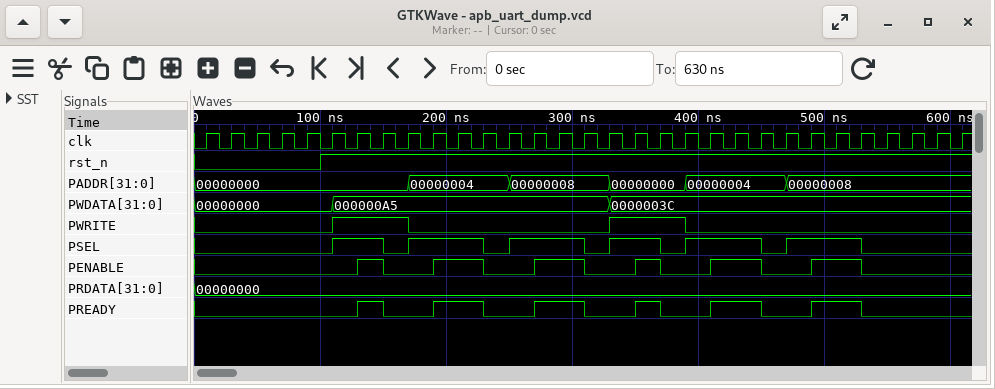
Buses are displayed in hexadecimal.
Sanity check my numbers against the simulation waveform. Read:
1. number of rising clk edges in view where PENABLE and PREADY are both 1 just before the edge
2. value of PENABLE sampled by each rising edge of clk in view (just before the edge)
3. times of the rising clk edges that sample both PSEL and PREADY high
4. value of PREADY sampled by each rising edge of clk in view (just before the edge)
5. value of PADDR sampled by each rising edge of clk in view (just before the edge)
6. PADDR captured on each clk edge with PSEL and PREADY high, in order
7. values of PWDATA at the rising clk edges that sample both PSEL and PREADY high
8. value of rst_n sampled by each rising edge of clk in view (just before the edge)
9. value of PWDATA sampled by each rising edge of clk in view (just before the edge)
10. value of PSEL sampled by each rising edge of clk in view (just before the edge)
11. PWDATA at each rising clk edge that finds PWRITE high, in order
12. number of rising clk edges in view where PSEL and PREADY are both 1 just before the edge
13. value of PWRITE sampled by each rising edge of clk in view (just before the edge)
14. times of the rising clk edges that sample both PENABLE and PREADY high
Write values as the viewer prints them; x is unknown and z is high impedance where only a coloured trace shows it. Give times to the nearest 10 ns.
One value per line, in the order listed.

10
0 0 0 0 0 0 0 1 0 0 1 1 0 0 1 1 0 0 1 0 0 1 1 0 0 1 1 0 0 0 0
150 ns, 210 ns, 230 ns, 290 ns, 310 ns, 370 ns, 430 ns, 450 ns, 510 ns, 530 ns
0 0 0 0 0 0 0 1 0 0 1 1 0 0 1 1 0 0 1 0 0 1 1 0 0 1 1 0 0 0 0
00000000, 00000000, 00000000, 00000000, 00000000, 00000000, 00000000, 00000000, 00000000, 00000004, 00000004, 00000004, 00000004, 00000008, 00000008, 00000008, 00000008, 00000000, 00000000, 00000000, 00000004, 00000004, 00000004, 00000004, 00000008, 00000008, 00000008, 00000008, 00000008, 00000008, 00000008
00000000, 00000004, 00000004, 00000008, 00000008, 00000000, 00000004, 00000004, 00000008, 00000008
000000A5, 000000A5, 000000A5, 000000A5, 000000A5, 0000003C, 0000003C, 0000003C, 0000003C, 0000003C
0 0 0 0 0 1 1 1 1 1 1 1 1 1 1 1 1 1 1 1 1 1 1 1 1 1 1 1 1 1 1
00000000, 00000000, 00000000, 00000000, 00000000, 00000000, 000000A5, 000000A5, 000000A5, 000000A5, 000000A5, 000000A5, 000000A5, 000000A5, 000000A5, 000000A5, 000000A5, 0000003C, 0000003C, 0000003C, 0000003C, 0000003C, 0000003C, 0000003C, 0000003C, 0000003C, 0000003C, 0000003C, 0000003C, 0000003C, 0000003C
0 0 0 0 0 0 1 1 0 1 1 1 0 1 1 1 0 1 1 0 1 1 1 0 1 1 1 0 0 0 0
000000A5, 000000A5, 000000A5, 0000003C, 0000003C, 0000003C
10
0 0 0 0 0 0 1 1 1 0 0 0 0 0 0 0 0 1 1 1 0 0 0 0 0 0 0 0 0 0 0
150 ns, 210 ns, 230 ns, 290 ns, 310 ns, 370 ns, 430 ns, 450 ns, 510 ns, 530 ns
